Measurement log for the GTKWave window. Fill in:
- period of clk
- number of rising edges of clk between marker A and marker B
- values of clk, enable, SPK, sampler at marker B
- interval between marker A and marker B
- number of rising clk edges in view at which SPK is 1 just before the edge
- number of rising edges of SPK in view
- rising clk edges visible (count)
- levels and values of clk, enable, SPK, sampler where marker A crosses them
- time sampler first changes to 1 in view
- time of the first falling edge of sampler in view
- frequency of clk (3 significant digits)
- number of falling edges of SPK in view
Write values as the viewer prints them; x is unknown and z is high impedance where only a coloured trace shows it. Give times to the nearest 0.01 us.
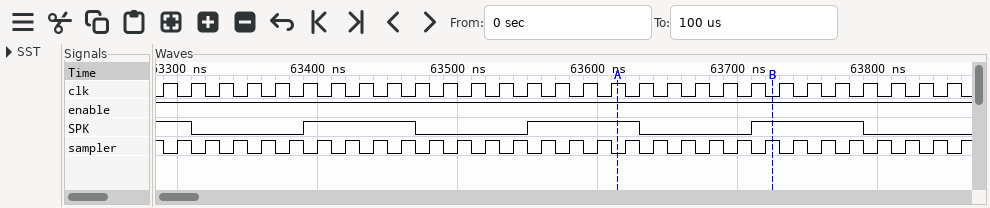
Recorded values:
0.02 us
5
clk=0, enable=1, SPK=1, sampler=1
0.11 us
14
3
29
clk=1, enable=1, SPK=1, sampler=0
63.3 us
63.29 us
50.0 MHz
4
